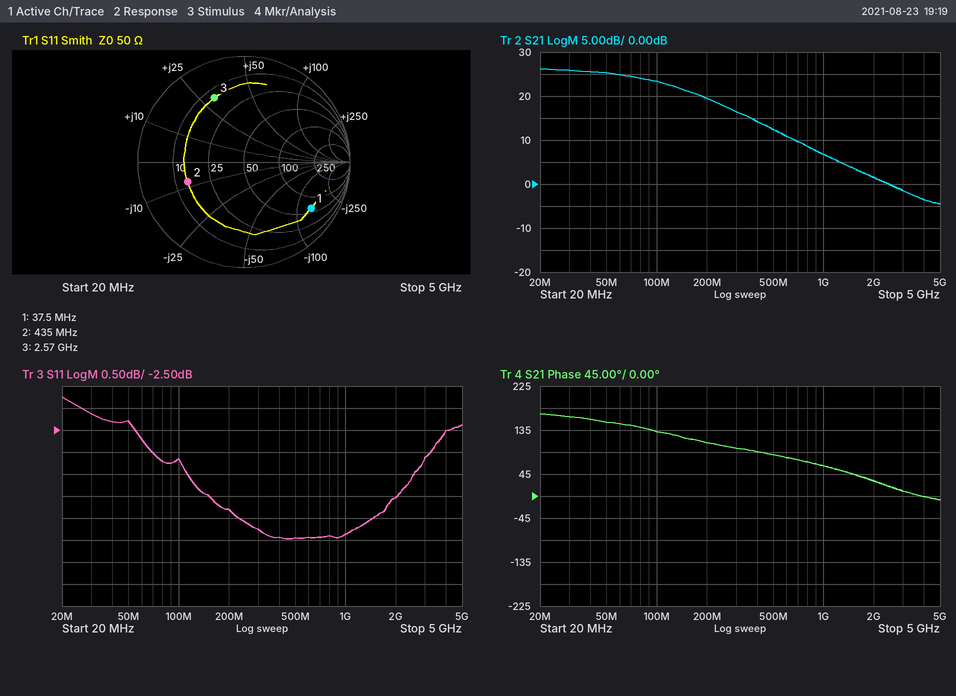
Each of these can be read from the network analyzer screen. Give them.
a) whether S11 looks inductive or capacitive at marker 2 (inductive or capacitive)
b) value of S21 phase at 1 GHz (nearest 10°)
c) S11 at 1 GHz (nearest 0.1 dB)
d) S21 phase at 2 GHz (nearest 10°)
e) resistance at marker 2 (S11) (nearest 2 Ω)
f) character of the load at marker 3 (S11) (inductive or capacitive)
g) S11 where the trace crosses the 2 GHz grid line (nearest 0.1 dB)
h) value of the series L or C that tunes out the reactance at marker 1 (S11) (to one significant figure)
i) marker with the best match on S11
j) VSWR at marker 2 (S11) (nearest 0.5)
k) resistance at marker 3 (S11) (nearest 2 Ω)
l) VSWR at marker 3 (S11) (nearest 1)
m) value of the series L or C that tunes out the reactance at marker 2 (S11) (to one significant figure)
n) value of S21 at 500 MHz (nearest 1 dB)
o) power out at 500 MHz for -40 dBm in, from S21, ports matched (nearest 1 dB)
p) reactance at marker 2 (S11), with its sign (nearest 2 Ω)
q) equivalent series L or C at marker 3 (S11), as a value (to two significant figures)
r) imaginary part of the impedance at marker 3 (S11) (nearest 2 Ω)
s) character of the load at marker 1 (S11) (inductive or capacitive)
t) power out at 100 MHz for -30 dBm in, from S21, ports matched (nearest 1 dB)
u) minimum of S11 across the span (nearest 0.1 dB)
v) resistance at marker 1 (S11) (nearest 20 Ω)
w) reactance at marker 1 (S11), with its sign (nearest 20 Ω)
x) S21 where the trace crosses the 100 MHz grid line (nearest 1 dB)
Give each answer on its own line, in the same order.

capacitive
60°
-4.9 dB
30°
14 Ω
inductive
-4.0 dB
600 nH
marker 2
3.5
14 Ω
5
3 nH
12 dB
-28 dBm
-8 Ω
1.9 nH
+30 Ω
capacitive
-7 dBm
-5.0 dB
60 Ω
-140 Ω
23 dB
